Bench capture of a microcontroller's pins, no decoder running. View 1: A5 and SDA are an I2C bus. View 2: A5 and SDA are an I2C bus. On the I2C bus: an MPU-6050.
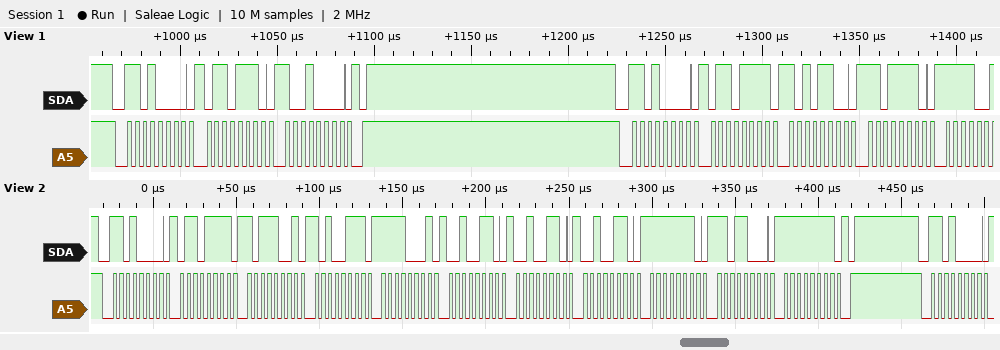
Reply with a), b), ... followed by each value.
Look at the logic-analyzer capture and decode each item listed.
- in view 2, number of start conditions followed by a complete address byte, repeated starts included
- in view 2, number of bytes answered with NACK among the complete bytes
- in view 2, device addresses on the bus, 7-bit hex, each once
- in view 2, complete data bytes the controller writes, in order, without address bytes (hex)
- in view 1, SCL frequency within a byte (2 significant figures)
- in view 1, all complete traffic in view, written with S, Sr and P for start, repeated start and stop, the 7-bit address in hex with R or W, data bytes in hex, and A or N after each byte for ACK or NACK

a) 2
b) 0
c) 0x68
d) 6F B9 A7 F1 26 26 26 FE D8 FF
e) 250 kHz
f) S 68W A 6E A 90 A P S 68W A 6F A AC A DE A
